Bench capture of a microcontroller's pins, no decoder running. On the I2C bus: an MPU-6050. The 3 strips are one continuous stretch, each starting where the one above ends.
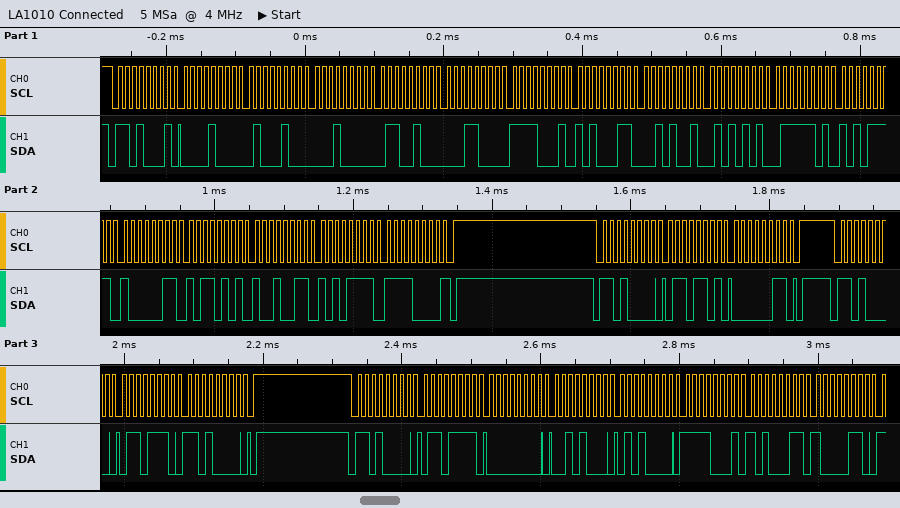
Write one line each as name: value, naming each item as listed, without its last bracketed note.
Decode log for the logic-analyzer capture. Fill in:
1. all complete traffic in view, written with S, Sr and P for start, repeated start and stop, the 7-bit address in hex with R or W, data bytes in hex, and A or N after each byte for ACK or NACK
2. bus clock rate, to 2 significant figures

all complete traffic in view, written with S, Sr and P for start, repeated start and stop, the 7-bit address in hex with R or W, data bytes in hex, and A or N after each byte for ACK or NACK: S 68R A 08 A 44 A 10 A 64 A 18 A F1 A A3 A 29 A 55 A 7D A AF A 83 A B5 A 93 A AF A F0 N P S 68W A 6D A 03 A P S 68W A 6E A D0 A P S 68W A 6F A 00 A 28 A 50 A F1 A A3 A 86 A
bus clock rate, to 2 significant figures: 100 kHz
